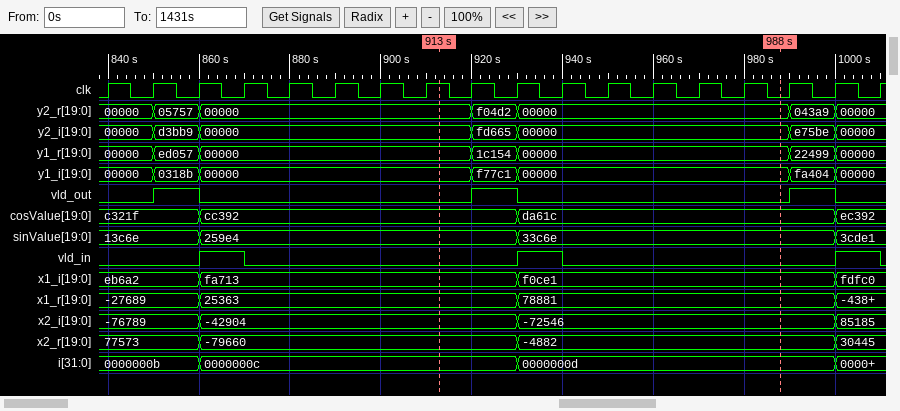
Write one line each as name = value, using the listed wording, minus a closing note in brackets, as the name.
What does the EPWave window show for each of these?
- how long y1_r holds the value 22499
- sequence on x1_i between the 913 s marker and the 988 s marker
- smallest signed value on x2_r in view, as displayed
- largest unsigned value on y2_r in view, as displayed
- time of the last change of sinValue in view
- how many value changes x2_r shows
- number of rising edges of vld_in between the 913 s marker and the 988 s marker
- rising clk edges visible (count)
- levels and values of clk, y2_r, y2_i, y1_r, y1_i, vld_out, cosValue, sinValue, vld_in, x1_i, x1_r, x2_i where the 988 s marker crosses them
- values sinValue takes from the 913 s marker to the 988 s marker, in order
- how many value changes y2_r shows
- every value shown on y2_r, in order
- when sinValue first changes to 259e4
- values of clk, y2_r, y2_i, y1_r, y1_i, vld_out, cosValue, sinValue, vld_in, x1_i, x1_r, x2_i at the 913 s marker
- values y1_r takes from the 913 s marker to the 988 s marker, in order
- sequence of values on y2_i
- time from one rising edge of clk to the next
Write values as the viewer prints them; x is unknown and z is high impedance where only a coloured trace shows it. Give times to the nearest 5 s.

how long y1_r holds the value 22499 = 10 s
sequence on x1_i between the 913 s marker and the 988 s marker = fa713, f0ce1
smallest signed value on x2_r in view, as displayed = -79660
largest unsigned value on y2_r in view, as displayed = f04d2
time of the last change of sinValue in view = 1000 s
how many value changes x2_r shows = 3
number of rising edges of vld_in between the 913 s marker and the 988 s marker = 1
rising clk edges visible = 18
levels and values of clk, y2_r, y2_i, y1_r, y1_i, vld_out, cosValue, sinValue, vld_in, x1_i, x1_r, x2_i where the 988 s marker crosses them = clk=0, y2_r=00000, y2_i=00000, y1_r=00000, y1_i=00000, vld_out=0, cosValue=da61c, sinValue=33c6e, vld_in=0, x1_i=f0ce1, x1_r=78881, x2_i=-72546
values sinValue takes from the 913 s marker to the 988 s marker, in order = 259e4, 33c6e
how many value changes y2_r shows = 6
every value shown on y2_r, in order = 00000, 05757, 00000, f04d2, 00000, 043a9, 00000
when sinValue first changes to 259e4 = 860 s
values of clk, y2_r, y2_i, y1_r, y1_i, vld_out, cosValue, sinValue, vld_in, x1_i, x1_r, x2_i at the 913 s marker = clk=1, y2_r=00000, y2_i=00000, y1_r=00000, y1_i=00000, vld_out=0, cosValue=cc392, sinValue=259e4, vld_in=0, x1_i=fa713, x1_r=25363, x2_i=-42904
values y1_r takes from the 913 s marker to the 988 s marker, in order = 00000, 1c154, 00000
sequence of values on y2_i = 00000, d3bb9, 00000, fd665, 00000, e75be, 00000
time from one rising edge of clk to the next = 10 s
